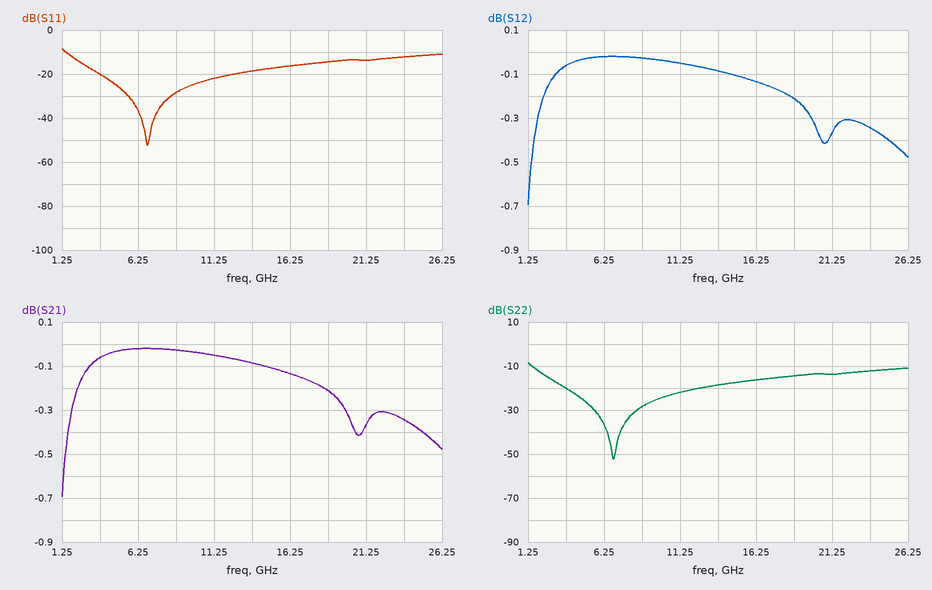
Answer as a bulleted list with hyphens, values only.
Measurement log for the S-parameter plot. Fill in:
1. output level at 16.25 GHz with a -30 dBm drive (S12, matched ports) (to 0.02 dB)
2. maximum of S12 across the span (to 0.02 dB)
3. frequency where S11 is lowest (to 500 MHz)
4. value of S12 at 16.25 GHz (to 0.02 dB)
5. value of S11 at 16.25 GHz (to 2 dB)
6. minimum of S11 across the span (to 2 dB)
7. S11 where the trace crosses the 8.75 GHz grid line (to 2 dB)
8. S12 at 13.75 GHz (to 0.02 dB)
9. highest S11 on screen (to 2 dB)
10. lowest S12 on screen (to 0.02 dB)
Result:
- -30.14 dBm
- -0.02 dB
- 7.0 GHz
- -0.14 dB
- -16 dB
- -52 dB
- -28 dB
- -0.08 dB
- -8 dB
- -0.70 dB
